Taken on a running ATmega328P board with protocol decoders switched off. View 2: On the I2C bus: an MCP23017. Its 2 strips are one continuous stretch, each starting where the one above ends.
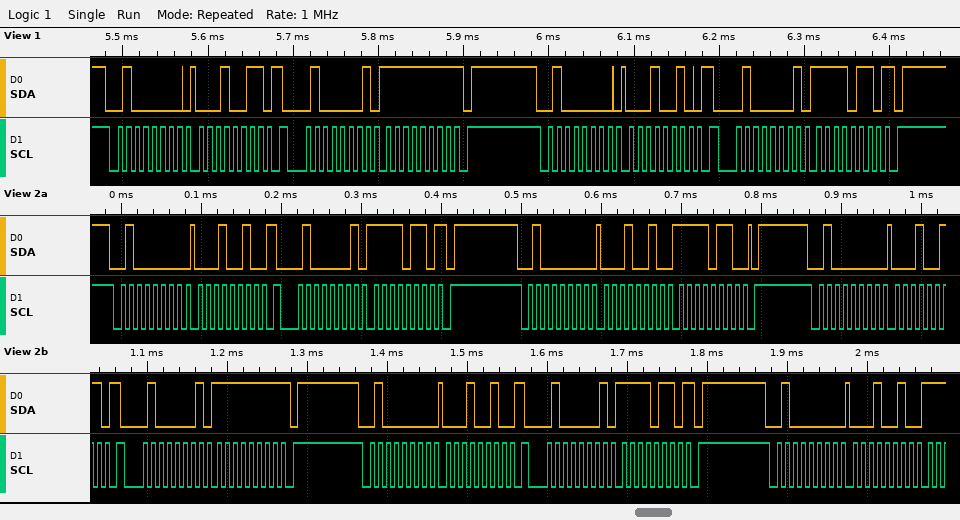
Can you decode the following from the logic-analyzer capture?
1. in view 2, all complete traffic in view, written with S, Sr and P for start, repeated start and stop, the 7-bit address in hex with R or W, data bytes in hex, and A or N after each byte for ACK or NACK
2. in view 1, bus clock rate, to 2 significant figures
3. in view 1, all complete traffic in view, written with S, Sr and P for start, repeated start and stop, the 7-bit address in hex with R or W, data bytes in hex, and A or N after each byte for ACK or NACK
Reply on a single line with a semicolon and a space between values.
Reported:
S 20W A 12 A Sr 20R A F6 N P S 20W A 12 A F6 A P S 20W A 13 A Sr 20R A FF N P S 20W A 12 A Sr 20R A F6 N P S 20W A 12 A; 100 kHz; S 20W A 13 A Sr 20R A FF N P S 20W A 12 A Sr 20R A F6 N P
